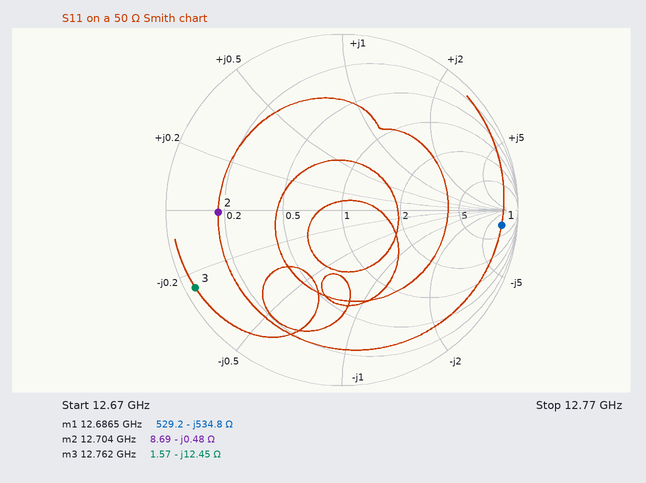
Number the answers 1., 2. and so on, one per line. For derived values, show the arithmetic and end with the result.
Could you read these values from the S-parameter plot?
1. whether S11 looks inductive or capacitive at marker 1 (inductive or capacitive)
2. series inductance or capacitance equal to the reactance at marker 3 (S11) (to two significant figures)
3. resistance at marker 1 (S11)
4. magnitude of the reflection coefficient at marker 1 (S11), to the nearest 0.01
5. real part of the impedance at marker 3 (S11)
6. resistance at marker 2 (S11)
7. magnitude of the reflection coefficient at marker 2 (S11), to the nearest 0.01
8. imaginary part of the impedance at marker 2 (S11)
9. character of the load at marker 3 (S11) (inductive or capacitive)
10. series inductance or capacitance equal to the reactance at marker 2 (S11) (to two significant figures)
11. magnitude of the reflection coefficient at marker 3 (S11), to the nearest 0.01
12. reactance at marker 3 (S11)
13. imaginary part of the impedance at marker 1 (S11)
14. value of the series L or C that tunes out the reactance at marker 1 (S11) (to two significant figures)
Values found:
1. capacitive
2. C = 1/(2π × 12.762 GHz × 12.45 Ω) ≈ 1.0 pF
3. 529.2 Ω
4. 0.91
5. 1.57 Ω
6. 8.69 Ω
7. 0.70
8. -0.48 Ω
9. capacitive
10. C = 1/(2π × 12.704 GHz × 0.48 Ω) ≈ 26 pF
11. 0.94
12. -12.45 Ω
13. -534.8 Ω
14. L = 534.8 Ω/(2π × 12.6865 GHz) ≈ 6.7 nH
